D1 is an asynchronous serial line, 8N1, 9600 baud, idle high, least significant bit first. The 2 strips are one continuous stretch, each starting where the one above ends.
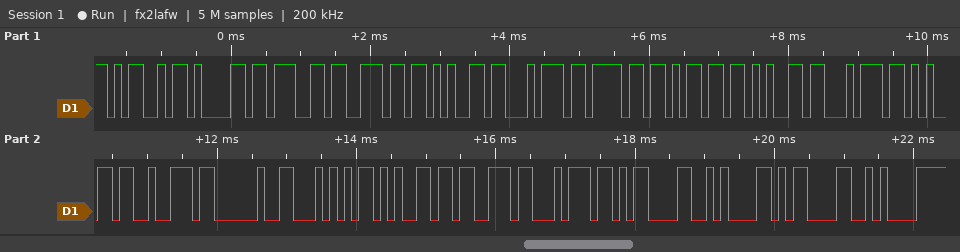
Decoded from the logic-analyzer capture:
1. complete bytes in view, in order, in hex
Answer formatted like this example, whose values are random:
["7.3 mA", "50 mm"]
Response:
["0x4D 0x61 0x67 0x6E 0x65 0x74 0x6F 0x6D 0x65 0x74 0x65 0x72 0x20 0x54 0x65 0x73 0x74 0x0D 0x0A 0x0D 0x0A"]
